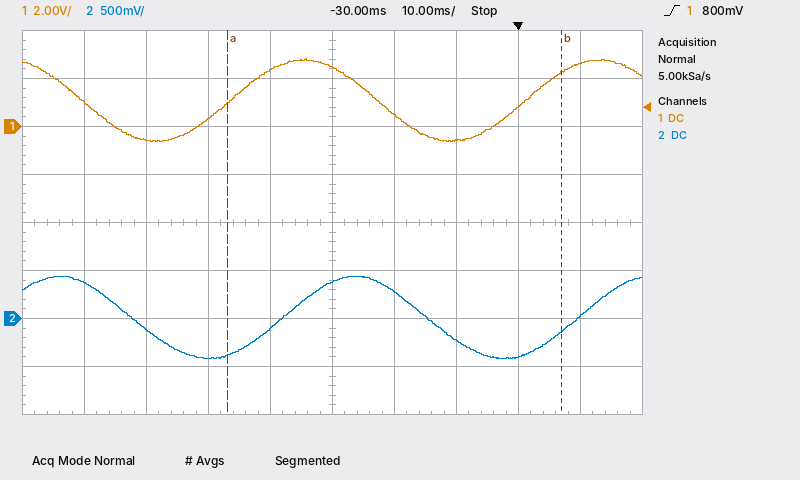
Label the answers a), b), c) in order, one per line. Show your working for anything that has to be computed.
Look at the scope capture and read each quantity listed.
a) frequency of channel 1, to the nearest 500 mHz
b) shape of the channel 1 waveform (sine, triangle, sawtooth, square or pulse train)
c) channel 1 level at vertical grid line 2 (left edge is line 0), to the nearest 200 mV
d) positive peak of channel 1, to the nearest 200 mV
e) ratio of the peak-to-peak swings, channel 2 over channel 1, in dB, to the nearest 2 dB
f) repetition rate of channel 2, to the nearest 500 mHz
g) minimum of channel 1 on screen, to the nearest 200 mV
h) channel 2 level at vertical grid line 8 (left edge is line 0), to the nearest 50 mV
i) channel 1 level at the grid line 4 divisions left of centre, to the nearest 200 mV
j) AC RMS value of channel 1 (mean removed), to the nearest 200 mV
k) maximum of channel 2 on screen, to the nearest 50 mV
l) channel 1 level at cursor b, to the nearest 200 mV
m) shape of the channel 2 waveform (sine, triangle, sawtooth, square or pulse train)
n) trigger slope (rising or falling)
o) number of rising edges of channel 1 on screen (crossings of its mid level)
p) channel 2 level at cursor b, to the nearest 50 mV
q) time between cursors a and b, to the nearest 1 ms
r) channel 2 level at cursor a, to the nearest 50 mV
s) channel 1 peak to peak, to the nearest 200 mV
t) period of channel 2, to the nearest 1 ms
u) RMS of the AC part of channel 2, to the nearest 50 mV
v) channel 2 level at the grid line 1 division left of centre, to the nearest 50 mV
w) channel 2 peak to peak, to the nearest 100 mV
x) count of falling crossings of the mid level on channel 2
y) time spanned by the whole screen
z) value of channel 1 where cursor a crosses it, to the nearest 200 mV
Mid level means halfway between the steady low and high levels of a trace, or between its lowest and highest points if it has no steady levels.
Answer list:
a) 21.0 Hz
b) sine
c) -600 mV
d) 2.8 V
e) 20 log10(900 mV / 3.4 V) ≈ -12 dB
f) 1 / 48 ms ≈ 20.8 Hz, so 21.0 Hz to the nearest 500 mHz
g) -600 mV
h) -400 mV
i) 1.0 V
j) 3.4 V / (2√2) ≈ 1.2 V
k) 450 mV
l) 2.2 V
m) sine
n) rising
o) 2
p) -150 mV
q) 54 ms
r) -400 mV
s) 2.8 V − (-600 mV) = 3.4 V
t) 48 ms
u) 900 mV / (2√2) ≈ 318 mV, so 300 mV to the nearest 50 mV
v) -100 mV
w) 900 mV
x) 2
y) 100 ms
z) 1.0 V
